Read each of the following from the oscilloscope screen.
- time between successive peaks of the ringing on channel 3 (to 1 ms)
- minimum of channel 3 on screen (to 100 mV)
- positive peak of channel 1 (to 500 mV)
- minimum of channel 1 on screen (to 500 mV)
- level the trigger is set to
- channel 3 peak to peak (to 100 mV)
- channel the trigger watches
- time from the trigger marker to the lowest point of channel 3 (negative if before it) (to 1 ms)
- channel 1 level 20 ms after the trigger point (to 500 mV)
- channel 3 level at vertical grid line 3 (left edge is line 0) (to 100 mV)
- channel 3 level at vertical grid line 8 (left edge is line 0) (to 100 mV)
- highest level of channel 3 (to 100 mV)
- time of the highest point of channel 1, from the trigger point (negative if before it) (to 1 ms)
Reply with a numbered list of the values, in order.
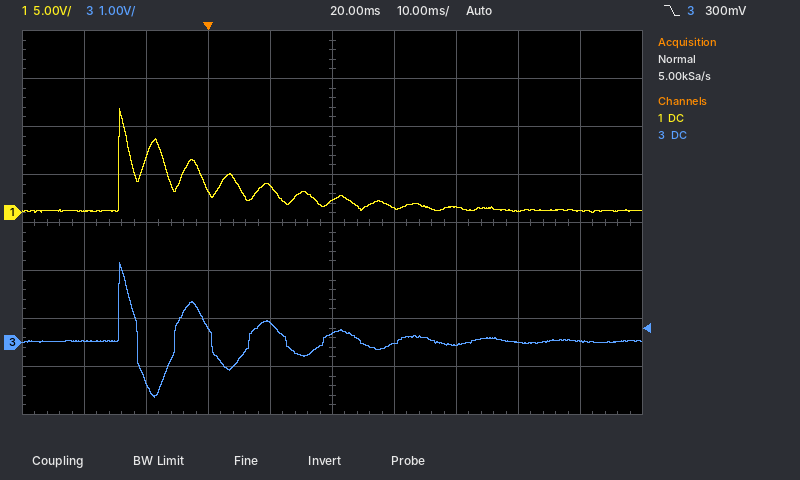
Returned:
1. 12 ms
2. -1.1 V
3. 11.0 V
4. 0.0 V
5. 300 mV
6. 2.8 V
7. channel 3
8. -9 ms
9. 1.5 V
10. 300 mV
11. 0.0 V
12. 1.7 V
13. -14 ms
